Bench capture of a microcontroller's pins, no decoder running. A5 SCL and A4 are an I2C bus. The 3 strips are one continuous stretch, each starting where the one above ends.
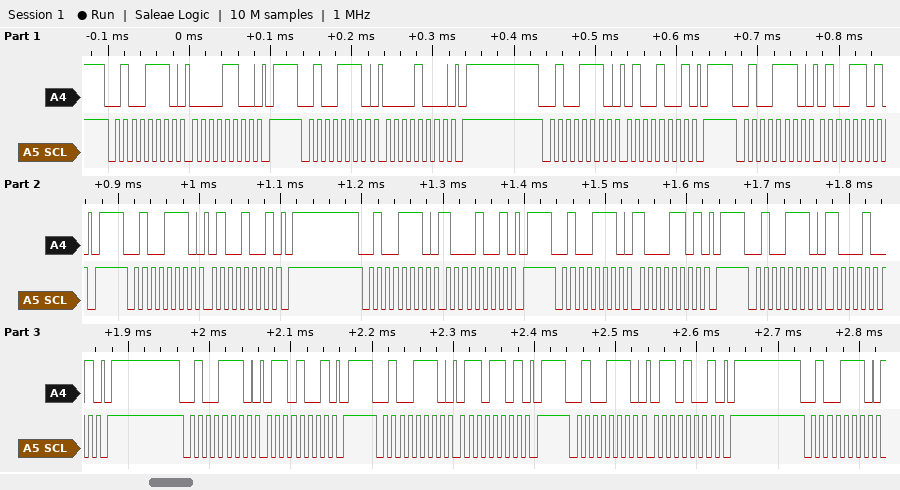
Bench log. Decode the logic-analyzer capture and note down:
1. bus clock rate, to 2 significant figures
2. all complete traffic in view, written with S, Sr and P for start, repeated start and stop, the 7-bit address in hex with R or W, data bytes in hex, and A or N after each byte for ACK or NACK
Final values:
100 kHz
S 27W A 0C A P S 27W A 08 A P S 27W A 49 A P S 27W A 4D A P S 27W A 49 A P S 27W A 89 A P S 27W A 8D A P S 27W A 89 A P S 27W A 69 A P S 27W A 6D A P S 27W A 69 A P S 27W A
